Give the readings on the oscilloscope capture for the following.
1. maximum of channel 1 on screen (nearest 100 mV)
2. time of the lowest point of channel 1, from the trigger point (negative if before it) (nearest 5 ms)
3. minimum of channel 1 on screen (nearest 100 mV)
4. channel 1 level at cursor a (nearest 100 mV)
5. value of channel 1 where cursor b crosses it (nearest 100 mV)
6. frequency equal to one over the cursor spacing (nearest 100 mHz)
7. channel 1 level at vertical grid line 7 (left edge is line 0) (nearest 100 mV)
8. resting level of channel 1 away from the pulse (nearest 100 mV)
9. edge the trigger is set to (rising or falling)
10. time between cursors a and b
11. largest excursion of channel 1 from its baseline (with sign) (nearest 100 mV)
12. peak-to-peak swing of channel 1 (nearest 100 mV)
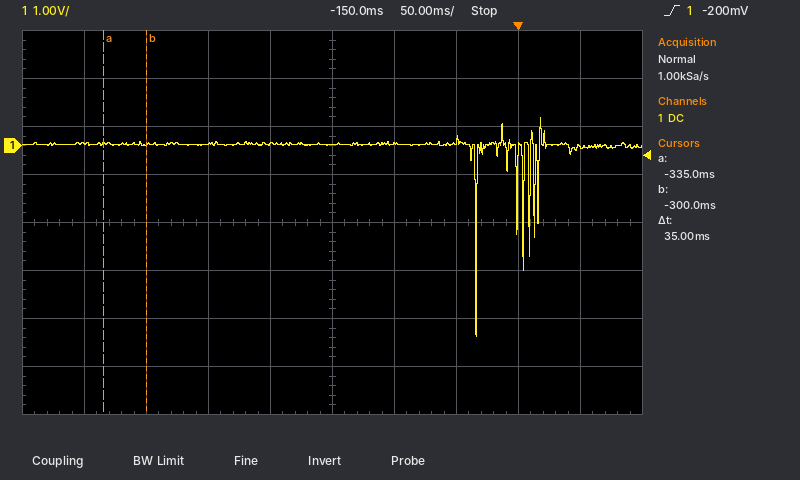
600 mV
-35 ms
-4.0 V
0.0 V
0.0 V
28.6 Hz
100 mV
0.0 V
rising
35 ms
-4.0 V
4.6 V
